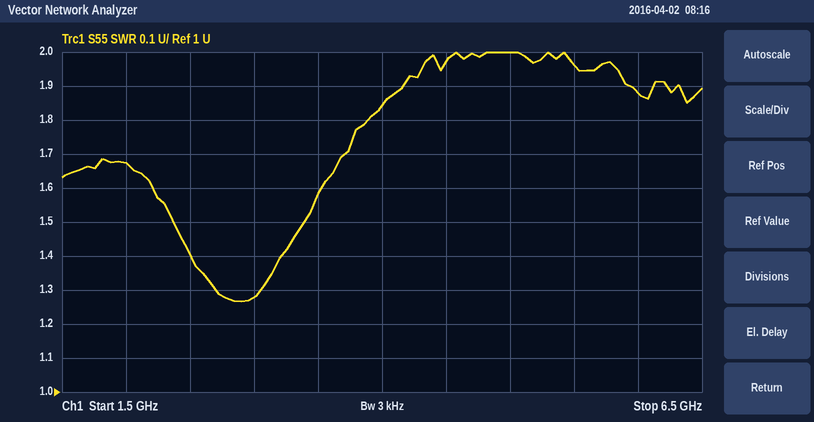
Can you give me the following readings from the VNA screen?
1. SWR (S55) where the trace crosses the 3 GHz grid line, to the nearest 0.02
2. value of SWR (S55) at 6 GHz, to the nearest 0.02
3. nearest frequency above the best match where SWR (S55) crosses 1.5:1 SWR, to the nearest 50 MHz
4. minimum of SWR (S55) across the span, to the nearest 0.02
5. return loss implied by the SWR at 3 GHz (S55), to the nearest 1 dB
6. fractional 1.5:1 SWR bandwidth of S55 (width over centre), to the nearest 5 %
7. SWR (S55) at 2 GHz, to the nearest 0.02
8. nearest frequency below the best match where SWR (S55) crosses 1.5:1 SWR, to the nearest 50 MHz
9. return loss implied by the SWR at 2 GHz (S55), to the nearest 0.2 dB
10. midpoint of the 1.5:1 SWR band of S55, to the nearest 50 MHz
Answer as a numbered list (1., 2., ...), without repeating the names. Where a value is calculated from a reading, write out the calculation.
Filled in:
1. 1.28
2. 1.88
3. 3.40 GHz
4. 1.26
5. −20 log10((1.28 − 1)/(1.28 + 1)) ≈ 18 dB
6. 1.05 GHz / 2.875 GHz ≈ 36.5 %, so 35 % to the nearest 5 %
7. 1.68
8. 2.35 GHz
9. −20 log10((1.68 − 1)/(1.68 + 1)) ≈ 11.9 dB, so 12.0 dB to the nearest 0.2 dB
10. 2.90 GHz
